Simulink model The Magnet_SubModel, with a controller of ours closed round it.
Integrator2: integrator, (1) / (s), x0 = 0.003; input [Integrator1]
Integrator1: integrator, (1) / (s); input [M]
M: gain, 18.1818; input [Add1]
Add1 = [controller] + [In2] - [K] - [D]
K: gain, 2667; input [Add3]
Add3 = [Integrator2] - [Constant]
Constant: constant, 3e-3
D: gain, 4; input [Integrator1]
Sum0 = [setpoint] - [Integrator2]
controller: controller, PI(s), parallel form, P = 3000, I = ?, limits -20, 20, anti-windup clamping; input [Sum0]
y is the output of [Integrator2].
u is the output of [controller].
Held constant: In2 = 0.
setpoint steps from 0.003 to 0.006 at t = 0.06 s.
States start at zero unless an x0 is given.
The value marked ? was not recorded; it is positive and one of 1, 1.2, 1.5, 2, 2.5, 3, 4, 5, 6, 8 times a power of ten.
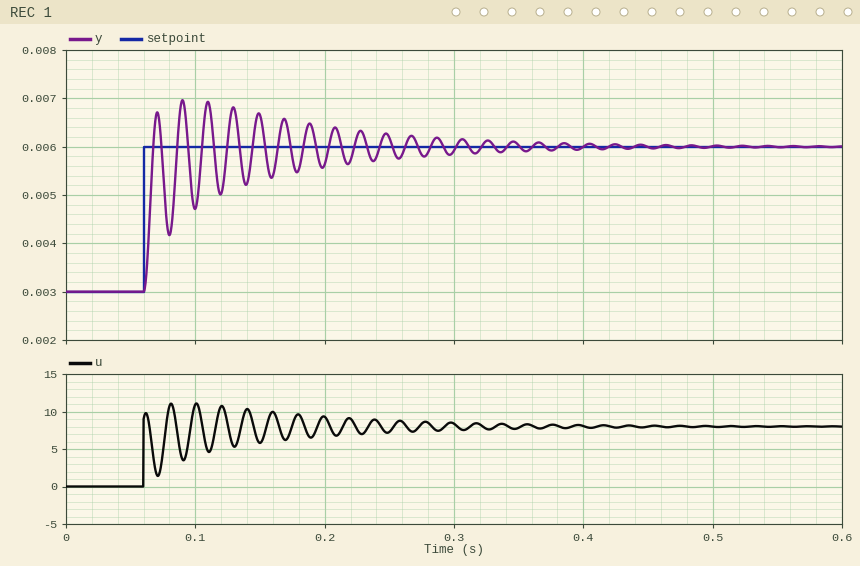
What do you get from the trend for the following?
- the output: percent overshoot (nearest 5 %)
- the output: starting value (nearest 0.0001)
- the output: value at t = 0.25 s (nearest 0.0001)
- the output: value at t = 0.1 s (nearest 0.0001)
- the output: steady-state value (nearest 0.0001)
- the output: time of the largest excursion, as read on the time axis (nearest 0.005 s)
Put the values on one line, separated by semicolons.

30 %; 0.0030; 0.0062; 0.0047; 0.0060; 0.090 s
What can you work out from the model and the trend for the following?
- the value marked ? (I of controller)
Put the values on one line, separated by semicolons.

300000
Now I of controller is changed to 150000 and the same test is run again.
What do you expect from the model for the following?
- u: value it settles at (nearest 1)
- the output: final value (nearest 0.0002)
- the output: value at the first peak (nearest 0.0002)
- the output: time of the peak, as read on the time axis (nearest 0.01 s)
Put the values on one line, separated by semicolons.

8; 0.0060; 0.0062; 0.07 s
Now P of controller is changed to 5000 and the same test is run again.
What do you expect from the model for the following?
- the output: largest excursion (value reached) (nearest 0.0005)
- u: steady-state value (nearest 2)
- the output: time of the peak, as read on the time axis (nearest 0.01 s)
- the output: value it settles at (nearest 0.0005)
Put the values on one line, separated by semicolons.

0.0070; 8; 0.07 s; 0.0060
